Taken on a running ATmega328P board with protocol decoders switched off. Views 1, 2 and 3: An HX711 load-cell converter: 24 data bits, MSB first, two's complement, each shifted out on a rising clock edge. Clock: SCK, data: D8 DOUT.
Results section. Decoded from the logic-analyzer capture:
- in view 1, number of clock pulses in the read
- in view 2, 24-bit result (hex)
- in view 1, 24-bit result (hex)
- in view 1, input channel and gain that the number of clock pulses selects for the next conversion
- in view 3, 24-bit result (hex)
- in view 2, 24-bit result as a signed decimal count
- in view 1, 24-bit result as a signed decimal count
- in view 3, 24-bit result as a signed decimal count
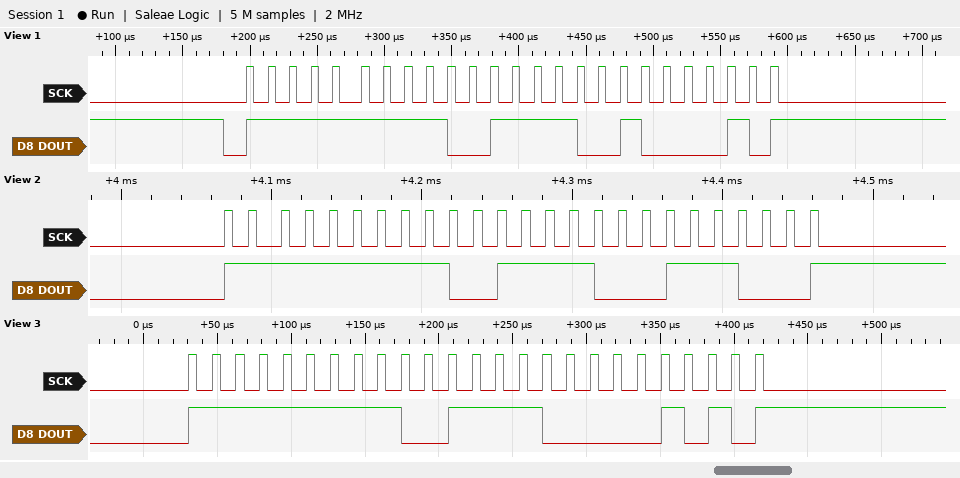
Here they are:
25
0xFF9E38
0xFF9E42
channel A, gain 128
0xFF9E0A
-25032
-25022
-25078
